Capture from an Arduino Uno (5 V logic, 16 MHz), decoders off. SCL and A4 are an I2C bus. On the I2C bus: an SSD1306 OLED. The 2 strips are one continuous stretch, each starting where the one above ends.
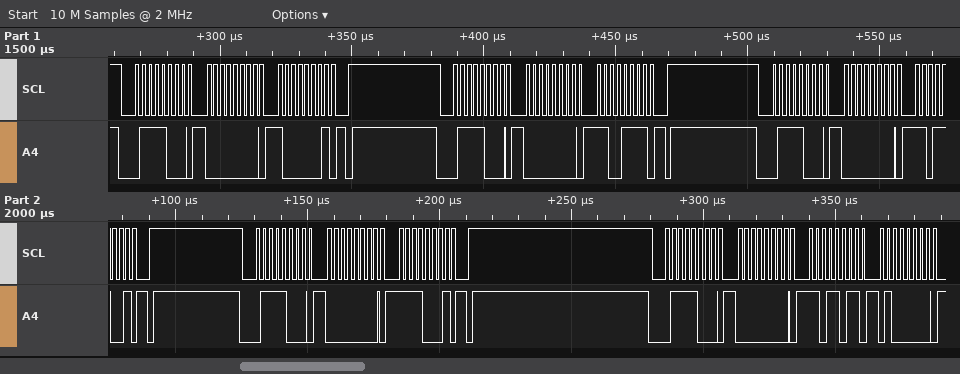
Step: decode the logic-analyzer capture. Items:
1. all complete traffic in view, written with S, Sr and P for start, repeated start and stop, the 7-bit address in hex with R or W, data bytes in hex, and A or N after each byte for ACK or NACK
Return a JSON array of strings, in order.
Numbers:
["S 3CW A 00 A 81 A P S 3CW A 00 A CF A P S 3CW A 00 A D9 A P S 3CW A 00 A F1 A P S 3CW A 00 A DB A 40 A"]
